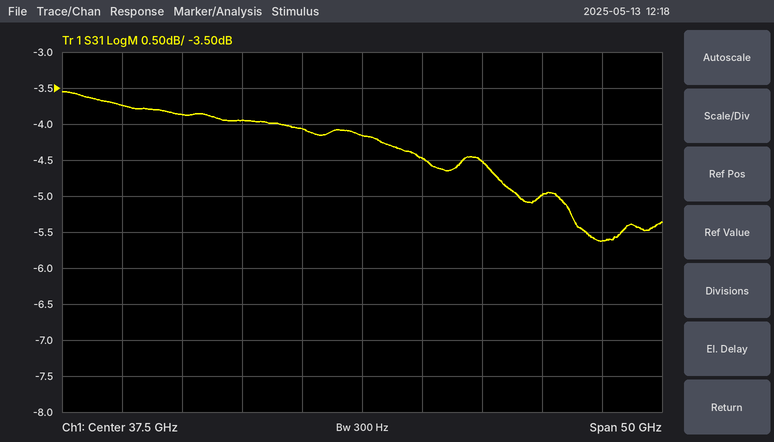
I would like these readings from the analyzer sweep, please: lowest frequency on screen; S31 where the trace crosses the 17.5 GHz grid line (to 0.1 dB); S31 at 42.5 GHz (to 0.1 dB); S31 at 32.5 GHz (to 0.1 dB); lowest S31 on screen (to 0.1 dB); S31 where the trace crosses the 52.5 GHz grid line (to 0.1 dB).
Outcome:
12.5 GHz
-3.7 dB
-4.5 dB
-4.1 dB
-5.6 dB
-5.0 dB
